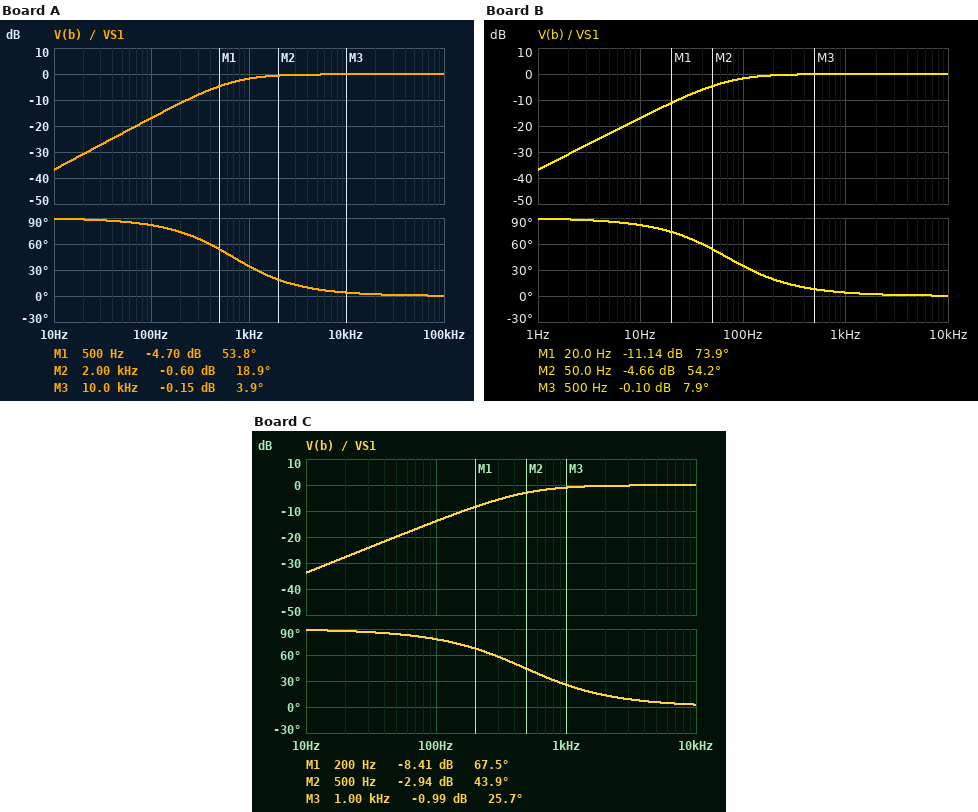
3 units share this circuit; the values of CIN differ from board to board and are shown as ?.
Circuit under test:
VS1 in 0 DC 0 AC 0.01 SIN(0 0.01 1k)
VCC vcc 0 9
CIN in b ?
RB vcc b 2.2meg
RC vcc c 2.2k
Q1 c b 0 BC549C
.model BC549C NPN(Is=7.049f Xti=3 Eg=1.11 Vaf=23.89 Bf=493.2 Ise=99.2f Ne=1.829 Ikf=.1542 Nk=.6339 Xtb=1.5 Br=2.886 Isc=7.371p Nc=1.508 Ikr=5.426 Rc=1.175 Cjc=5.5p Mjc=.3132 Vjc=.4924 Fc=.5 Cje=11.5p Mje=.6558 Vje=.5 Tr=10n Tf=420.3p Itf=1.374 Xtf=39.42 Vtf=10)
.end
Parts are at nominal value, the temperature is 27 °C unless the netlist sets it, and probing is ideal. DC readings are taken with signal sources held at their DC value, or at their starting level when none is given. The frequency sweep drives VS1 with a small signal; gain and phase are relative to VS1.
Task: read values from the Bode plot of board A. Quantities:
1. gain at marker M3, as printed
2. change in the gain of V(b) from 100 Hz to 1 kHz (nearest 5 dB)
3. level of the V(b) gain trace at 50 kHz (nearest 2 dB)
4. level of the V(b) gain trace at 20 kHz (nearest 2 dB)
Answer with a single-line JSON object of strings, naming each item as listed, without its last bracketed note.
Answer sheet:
{"gain at marker M3, as printed": "-0.15 dB", "change in the gain of V(b) from 100 Hz to 1 kHz": "15 dB", "level of the V(b) gain trace at 50 kHz": "0 dB", "level of the V(b) gain trace at 20 kHz": "0 dB"}
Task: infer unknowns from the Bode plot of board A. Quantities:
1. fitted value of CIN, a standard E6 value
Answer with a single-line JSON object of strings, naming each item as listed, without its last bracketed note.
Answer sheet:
{"fitted value of CIN, a standard E6 value": "33 nF"}
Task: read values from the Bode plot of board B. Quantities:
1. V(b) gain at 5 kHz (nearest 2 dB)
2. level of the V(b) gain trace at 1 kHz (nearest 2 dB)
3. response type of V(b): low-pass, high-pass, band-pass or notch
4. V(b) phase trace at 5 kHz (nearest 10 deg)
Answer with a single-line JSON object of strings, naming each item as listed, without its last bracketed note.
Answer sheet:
{"V(b) gain at 5 kHz": "0 dB", "level of the V(b) gain trace at 1 kHz": "0 dB", "response type of V(b): low-pass, high-pass, band-pass or notch": "high-pass", "V(b) phase trace at 5 kHz": "0 deg"}
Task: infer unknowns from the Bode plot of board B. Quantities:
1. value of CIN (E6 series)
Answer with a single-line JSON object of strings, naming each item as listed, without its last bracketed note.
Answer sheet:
{"value of CIN": "330 nF"}
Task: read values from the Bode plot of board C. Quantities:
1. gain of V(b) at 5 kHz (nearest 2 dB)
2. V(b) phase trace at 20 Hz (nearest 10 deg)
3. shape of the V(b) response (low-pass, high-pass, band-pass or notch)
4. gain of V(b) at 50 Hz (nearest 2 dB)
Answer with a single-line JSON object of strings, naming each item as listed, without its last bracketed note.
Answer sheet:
{"gain of V(b) at 5 kHz": "0 dB", "V(b) phase trace at 20 Hz": "90 deg", "shape of the V(b) response": "high-pass", "gain of V(b) at 50 Hz": "-20 dB"}
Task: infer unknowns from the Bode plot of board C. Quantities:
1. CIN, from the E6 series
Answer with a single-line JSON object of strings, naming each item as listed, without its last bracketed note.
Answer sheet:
{"CIN, from the E6 series": "47 nF"}
